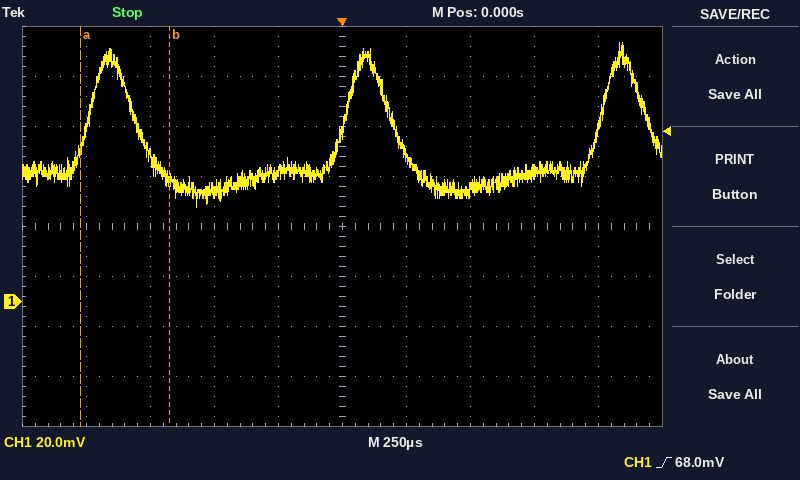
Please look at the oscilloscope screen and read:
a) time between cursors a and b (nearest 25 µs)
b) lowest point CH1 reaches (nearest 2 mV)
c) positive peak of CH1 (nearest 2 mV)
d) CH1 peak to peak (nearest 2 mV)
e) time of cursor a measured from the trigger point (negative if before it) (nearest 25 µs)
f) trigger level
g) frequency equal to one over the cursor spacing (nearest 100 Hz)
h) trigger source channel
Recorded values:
350 µs
38 mV
104 mV
66 mV
-1.025 ms
68.0 mV
2.9 kHz
CH1
